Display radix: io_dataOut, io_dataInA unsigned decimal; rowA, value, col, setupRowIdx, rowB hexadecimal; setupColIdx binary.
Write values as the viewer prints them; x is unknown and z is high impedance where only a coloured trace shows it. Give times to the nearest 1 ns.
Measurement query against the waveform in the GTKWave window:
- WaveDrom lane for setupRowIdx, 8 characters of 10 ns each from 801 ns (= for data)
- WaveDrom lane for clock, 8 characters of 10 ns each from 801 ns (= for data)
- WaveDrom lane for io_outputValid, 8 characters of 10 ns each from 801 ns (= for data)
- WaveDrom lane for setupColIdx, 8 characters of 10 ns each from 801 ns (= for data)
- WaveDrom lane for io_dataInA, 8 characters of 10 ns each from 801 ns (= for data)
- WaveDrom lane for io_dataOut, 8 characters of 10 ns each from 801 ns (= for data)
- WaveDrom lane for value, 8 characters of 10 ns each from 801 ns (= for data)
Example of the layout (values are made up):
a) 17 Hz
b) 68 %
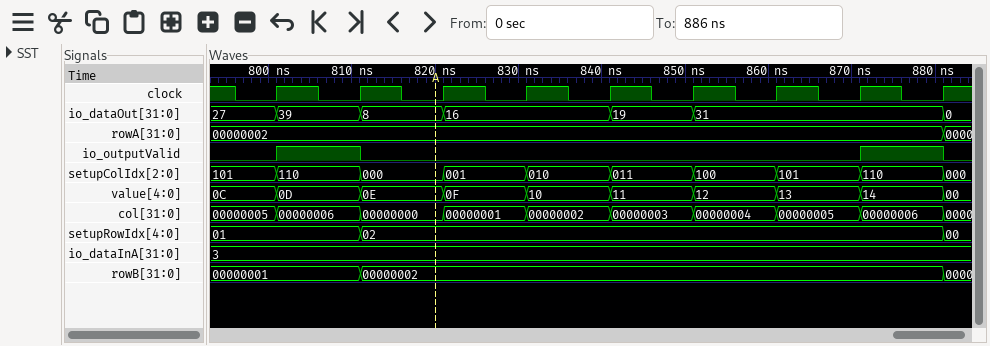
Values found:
a) {name: 'setupRowIdx', wave: '==......', data: '01 02'}
b) {name: 'clock', wave: 'p.......'}
c) {name: 'io_outputValid', wave: '10.....1'}
d) {name: 'setupColIdx', wave: '========', data: '110 000 001 010 011 100 101 110'}
e) {name: 'io_dataInA', wave: '=.......', data: '3'}
f) {name: 'io_dataOut', wave: '===.==..', data: '39 8 16 19 31'}
g) {name: 'value', wave: '========', data: '0D 0E 0F 10 11 12 13 14'}
